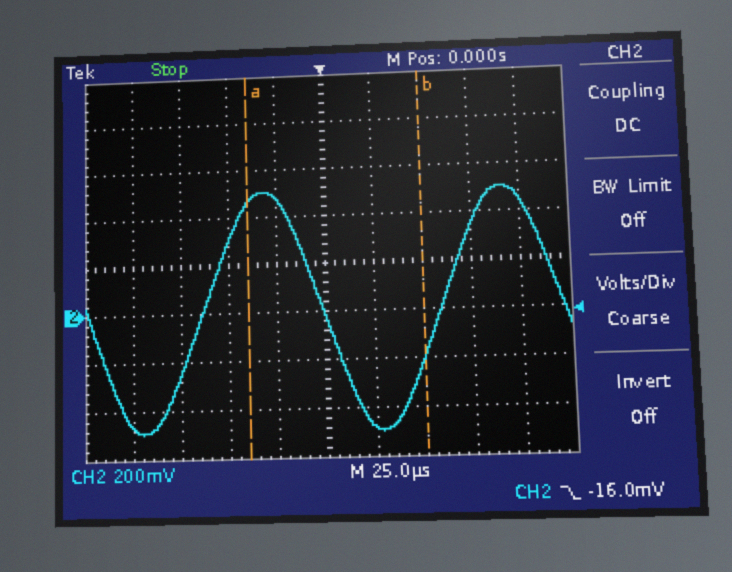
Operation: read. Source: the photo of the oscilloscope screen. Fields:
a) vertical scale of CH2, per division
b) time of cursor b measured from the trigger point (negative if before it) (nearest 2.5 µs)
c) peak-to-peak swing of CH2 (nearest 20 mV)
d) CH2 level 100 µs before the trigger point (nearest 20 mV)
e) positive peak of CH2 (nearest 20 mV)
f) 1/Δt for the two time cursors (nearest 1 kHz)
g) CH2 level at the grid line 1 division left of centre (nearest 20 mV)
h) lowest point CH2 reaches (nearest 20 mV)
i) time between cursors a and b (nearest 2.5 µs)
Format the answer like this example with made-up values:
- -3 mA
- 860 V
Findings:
- 200 mV
- +50.0 µs
- 1.00 V
- -460 mV
- 500 mV
- 11 kHz
- 480 mV
- -500 mV
- 90.0 µs
